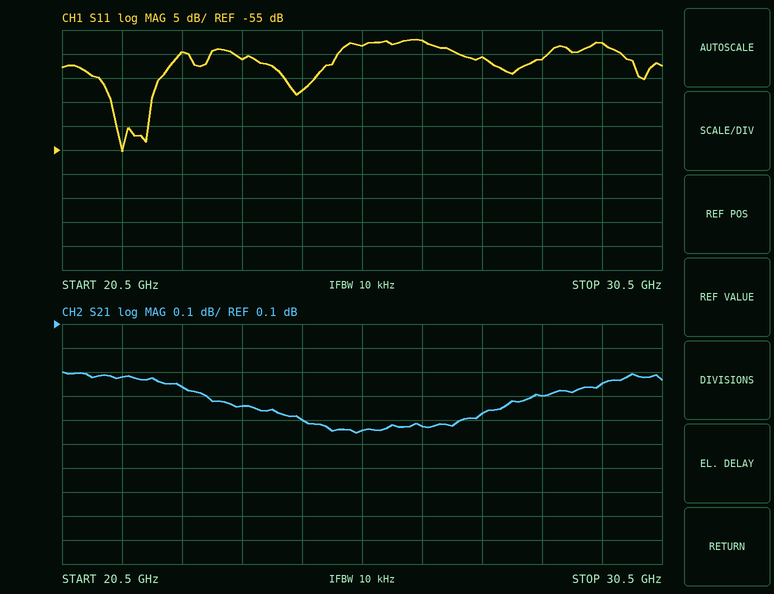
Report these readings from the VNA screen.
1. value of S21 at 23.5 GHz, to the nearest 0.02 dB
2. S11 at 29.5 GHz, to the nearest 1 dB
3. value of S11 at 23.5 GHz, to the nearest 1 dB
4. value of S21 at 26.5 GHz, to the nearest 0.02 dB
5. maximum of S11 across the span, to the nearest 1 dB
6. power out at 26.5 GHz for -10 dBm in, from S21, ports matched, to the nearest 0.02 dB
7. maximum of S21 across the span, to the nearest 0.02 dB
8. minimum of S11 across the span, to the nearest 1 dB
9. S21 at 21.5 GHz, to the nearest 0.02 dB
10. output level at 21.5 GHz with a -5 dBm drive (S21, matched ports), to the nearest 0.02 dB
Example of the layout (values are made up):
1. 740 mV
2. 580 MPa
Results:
1. -0.24 dB
2. -33 dB
3. -36 dB
4. -0.32 dB
5. -32 dB
6. -10.32 dBm
7. -0.10 dB
8. -55 dB
9. -0.12 dB
10. -5.12 dBm
